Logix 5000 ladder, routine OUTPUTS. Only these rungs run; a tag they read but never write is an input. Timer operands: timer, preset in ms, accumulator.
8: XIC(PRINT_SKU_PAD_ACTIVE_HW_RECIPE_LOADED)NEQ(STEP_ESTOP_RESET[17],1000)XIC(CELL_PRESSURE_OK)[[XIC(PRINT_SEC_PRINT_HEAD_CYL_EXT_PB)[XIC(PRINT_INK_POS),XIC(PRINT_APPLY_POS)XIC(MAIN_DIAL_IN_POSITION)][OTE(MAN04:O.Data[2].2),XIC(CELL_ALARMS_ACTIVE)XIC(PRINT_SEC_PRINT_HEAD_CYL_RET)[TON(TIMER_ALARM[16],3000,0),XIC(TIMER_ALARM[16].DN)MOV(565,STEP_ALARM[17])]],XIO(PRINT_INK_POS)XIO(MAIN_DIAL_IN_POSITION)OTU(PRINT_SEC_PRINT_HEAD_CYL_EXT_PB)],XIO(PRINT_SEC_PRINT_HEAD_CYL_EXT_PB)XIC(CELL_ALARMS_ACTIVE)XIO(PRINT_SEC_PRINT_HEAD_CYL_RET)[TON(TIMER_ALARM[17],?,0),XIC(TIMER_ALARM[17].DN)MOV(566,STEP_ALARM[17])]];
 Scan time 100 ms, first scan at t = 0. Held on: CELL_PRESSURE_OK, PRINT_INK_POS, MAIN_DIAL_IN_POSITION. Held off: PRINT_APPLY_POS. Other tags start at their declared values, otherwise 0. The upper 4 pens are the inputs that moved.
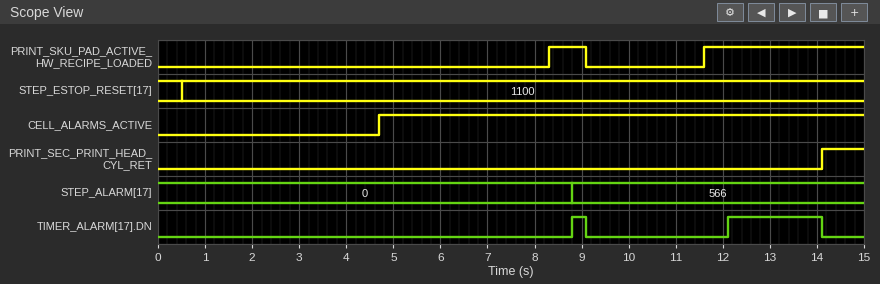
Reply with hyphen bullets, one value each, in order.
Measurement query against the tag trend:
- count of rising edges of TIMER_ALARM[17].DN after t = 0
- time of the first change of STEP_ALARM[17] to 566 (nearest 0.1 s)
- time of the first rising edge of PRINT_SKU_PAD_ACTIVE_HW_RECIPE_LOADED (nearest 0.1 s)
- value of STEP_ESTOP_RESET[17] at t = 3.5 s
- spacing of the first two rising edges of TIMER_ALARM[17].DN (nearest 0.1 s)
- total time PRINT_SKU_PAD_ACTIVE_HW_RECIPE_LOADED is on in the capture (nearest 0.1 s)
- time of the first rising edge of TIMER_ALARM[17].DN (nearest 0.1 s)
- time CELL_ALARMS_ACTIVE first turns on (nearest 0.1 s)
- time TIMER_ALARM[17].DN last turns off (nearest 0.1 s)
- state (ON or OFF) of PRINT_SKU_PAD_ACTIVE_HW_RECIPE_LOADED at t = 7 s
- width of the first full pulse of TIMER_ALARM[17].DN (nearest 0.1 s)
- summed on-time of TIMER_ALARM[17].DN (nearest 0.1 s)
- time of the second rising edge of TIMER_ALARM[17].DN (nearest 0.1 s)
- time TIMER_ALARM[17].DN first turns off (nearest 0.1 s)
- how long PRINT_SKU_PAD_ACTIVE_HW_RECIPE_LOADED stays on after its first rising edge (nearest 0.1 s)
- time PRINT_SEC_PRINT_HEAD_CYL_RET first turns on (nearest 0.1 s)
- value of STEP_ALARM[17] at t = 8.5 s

- 2
- 8.8 s
- 8.3 s
- 1100
- 3.3 s
- 4.2 s
- 8.8 s
- 4.7 s
- 14.1 s
- OFF
- 0.3 s
- 2.3 s
- 12.1 s
- 9.1 s
- 0.8 s
- 14.1 s
- 0
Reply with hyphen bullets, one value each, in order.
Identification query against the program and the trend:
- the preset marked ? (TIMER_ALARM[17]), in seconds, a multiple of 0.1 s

- 0.5 s
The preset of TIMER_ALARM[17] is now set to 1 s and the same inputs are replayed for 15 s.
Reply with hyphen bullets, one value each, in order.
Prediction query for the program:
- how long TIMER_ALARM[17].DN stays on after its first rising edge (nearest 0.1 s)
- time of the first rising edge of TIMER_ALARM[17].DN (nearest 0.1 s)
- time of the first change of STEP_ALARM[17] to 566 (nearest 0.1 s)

- 1.5 s
- 12.6 s
- 12.6 s
